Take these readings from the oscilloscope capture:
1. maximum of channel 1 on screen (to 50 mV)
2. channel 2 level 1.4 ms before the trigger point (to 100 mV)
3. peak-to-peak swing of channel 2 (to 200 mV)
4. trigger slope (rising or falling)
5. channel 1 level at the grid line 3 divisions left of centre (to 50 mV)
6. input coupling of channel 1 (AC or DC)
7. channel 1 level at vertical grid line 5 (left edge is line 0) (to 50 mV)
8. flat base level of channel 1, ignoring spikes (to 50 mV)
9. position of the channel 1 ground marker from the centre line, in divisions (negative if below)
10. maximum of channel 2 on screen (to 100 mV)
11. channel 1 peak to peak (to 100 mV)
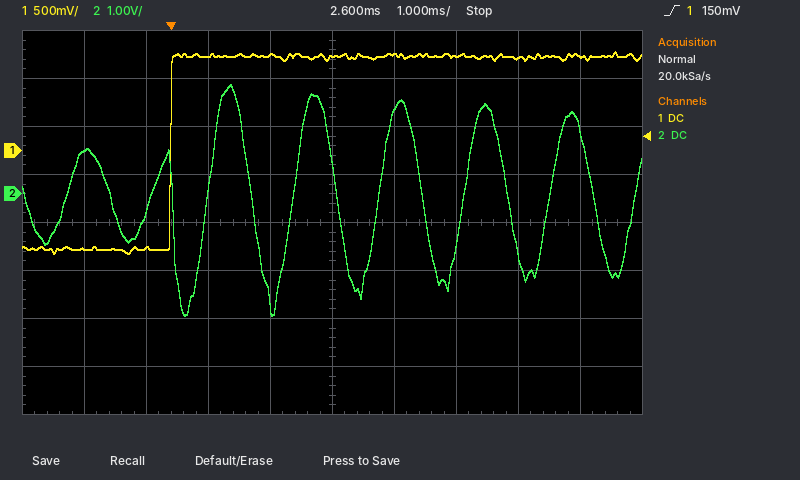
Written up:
1.05 V
900 mV
4.8 V
rising
-1.00 V
DC
1.00 V
-1.05 V
+1.5 div
2.3 V
2.10 V
